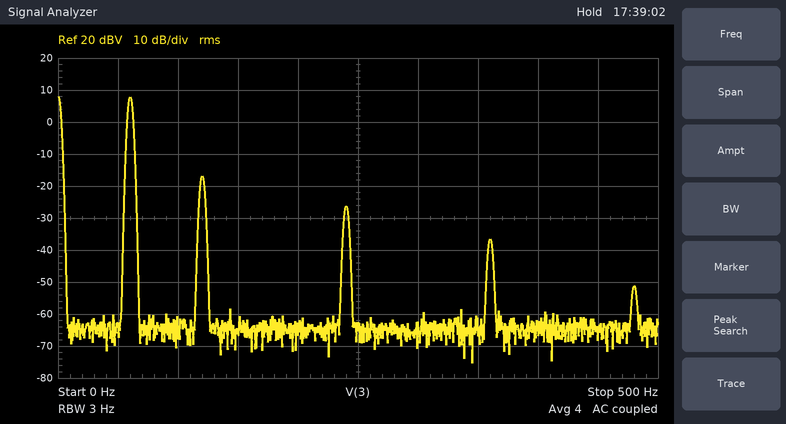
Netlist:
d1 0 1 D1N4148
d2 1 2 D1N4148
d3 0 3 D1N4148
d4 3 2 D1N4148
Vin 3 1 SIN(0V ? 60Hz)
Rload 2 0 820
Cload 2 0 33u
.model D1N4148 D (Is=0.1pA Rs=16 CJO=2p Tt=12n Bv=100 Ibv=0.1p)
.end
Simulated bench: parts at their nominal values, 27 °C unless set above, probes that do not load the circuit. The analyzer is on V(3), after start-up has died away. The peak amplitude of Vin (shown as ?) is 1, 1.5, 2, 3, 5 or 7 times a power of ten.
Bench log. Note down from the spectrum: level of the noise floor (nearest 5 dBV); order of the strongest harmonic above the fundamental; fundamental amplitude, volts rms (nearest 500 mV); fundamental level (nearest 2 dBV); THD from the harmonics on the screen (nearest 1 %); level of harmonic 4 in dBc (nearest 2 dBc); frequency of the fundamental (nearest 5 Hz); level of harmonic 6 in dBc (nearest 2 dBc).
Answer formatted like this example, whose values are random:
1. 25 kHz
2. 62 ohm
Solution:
1. -65 dBV
2. 2
3. 2.5 V
4. 8 dBV
5. 6 %
6. -34 dBc
7. 60 Hz
8. -44 dBc
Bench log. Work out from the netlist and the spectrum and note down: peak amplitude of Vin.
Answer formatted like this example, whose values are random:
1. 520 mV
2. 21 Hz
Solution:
1. 7 V
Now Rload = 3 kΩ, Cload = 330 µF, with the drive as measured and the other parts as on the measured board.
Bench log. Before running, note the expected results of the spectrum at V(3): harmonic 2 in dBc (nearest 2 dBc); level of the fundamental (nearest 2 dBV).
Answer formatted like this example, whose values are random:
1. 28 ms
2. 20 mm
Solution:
1. -54 dBc
2. 8 dBV
